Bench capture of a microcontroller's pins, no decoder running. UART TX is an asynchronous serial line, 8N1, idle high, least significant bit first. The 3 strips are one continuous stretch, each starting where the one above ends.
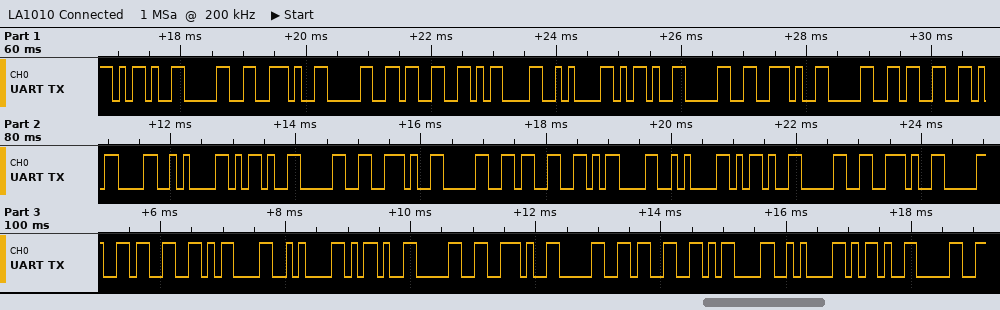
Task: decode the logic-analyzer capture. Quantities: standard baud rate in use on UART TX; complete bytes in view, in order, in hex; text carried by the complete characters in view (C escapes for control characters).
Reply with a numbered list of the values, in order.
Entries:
1. 9600 baud
2. 0x2D 0x30 0x2E 0x30 0x33 0x0D 0x0A 0x2D 0x30 0x2E 0x30 0x33 0x0D 0x0A 0x2D 0x30 0x2E 0x30 0x33 0x0D 0x0A 0x2D 0x30 0x2E 0x30 0x33 0x0D 0x0A 0x2D 0x30 0x2E 0x30 0x33 0x0D 0x0A 0x2D 0x30
3. "-0.03\r\n-0.03\r\n-0.03\r\n-0.03\r\n-0.03\r\n-0"
